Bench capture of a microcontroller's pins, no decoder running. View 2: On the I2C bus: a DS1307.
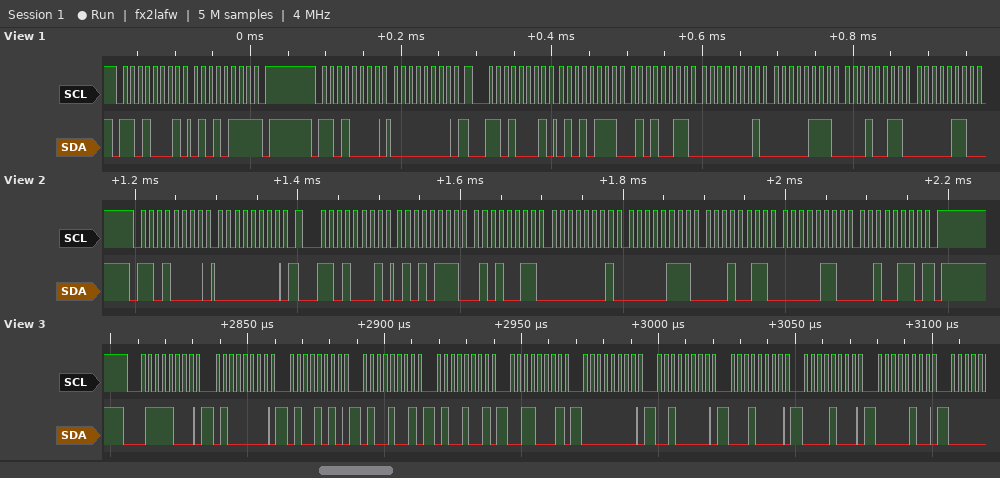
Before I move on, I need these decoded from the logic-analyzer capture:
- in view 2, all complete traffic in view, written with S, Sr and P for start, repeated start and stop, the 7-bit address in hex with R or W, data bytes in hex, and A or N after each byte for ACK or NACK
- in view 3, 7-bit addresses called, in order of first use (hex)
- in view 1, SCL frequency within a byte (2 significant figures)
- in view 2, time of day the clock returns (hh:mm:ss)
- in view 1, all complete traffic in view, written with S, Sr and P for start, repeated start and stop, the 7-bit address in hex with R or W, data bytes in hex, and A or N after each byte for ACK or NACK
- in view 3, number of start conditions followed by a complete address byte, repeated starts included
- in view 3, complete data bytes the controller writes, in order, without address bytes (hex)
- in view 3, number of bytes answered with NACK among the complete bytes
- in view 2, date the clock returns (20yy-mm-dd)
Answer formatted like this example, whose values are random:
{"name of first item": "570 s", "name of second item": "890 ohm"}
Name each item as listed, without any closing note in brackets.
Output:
{"in view 2, all complete traffic in view, written with S, Sr and P for start, repeated start and stop, the 7-bit address in hex with R or W, data bytes in hex, and A or N after each byte for ACK or NACK": "S 68W A 00 A Sr 68R A 57 A 53 A 01 A 07 A 13 A 06 A 26 N P", "in view 3, 7-bit addresses called, in order of first use": "0x3C", "in view 1, SCL frequency within a byte": "100 kHz", "in view 2, time of day the clock returns": "01:53:57", "in view 1, all complete traffic in view, written with S, Sr and P for start, repeated start and stop, the 7-bit address in hex with R or W, data bytes in hex, and A or N after each byte for ACK or NACK": "S 68R A 57 N P S 68W A 00 A Sr 68R A 57 A 53 A 01 A 07 A 13 A 06 A", "in view 3, number of start conditions followed by a complete address byte, repeated starts included": "1", "in view 3, complete data bytes the controller writes, in order, without address bytes": "40 4A 49 49 31 00 20 10 08 04", "in view 3, number of bytes answered with NACK among the complete bytes": "0", "in view 2, date the clock returns": "2026-06-13"}
